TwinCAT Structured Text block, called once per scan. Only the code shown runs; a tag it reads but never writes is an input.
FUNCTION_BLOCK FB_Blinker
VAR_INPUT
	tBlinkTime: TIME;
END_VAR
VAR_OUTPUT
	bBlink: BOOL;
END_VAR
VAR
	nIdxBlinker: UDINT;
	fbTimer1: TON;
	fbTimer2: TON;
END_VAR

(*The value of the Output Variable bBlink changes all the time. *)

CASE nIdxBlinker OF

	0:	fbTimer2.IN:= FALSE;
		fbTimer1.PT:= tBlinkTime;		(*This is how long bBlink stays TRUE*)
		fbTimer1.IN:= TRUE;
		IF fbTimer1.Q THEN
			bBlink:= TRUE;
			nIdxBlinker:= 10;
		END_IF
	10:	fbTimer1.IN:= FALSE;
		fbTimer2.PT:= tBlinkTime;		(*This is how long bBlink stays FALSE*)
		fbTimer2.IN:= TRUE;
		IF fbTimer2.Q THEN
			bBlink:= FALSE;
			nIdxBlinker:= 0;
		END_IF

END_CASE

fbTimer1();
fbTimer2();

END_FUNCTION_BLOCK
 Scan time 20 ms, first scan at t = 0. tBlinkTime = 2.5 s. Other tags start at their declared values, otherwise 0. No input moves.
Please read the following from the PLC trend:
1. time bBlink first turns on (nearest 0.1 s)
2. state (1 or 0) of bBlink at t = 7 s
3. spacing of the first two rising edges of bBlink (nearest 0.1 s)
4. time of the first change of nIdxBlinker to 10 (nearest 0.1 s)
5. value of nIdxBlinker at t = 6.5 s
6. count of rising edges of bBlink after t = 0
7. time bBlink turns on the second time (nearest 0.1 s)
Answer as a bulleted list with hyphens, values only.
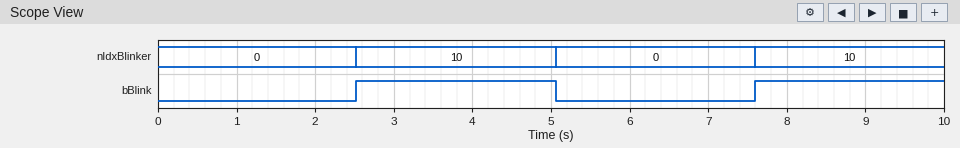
- 2.5 s
- 0
- 5.1 s
- 2.5 s
- 0
- 2
- 7.6 s
